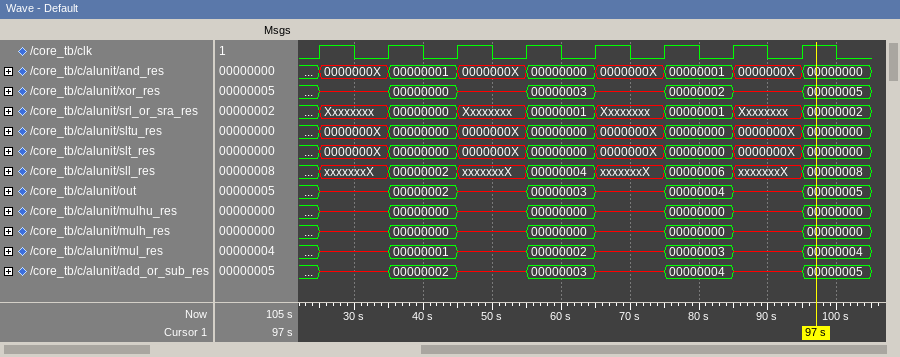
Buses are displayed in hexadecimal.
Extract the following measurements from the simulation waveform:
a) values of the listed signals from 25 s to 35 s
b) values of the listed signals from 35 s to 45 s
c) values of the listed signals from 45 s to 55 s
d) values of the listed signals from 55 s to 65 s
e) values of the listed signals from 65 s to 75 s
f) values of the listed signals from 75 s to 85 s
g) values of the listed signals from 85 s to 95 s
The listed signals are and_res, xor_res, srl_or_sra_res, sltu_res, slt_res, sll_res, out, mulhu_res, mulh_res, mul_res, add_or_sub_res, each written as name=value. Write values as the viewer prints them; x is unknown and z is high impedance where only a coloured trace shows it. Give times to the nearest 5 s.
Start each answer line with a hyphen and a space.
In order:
- and_res=0000000X, xor_res=x, srl_or_sra_res=Xxxxxxxx, sltu_res=0000000X, slt_res=0000000X, sll_res=xxxxxxxX, out=x, mulhu_res=x, mulh_res=x, mul_res=x, add_or_sub_res=x
- and_res=00000001, xor_res=00000000, srl_or_sra_res=00000000, sltu_res=00000000, slt_res=00000000, sll_res=00000002, out=00000002, mulhu_res=00000000, mulh_res=00000000, mul_res=00000001, add_or_sub_res=00000002
- and_res=0000000X, xor_res=x, srl_or_sra_res=Xxxxxxxx, sltu_res=0000000X, slt_res=0000000X, sll_res=xxxxxxxX, out=x, mulhu_res=x, mulh_res=x, mul_res=x, add_or_sub_res=x
- and_res=00000000, xor_res=00000003, srl_or_sra_res=00000001, sltu_res=00000000, slt_res=00000000, sll_res=00000004, out=00000003, mulhu_res=00000000, mulh_res=00000000, mul_res=00000002, add_or_sub_res=00000003
- and_res=0000000X, xor_res=x, srl_or_sra_res=Xxxxxxxx, sltu_res=0000000X, slt_res=0000000X, sll_res=xxxxxxxX, out=x, mulhu_res=x, mulh_res=x, mul_res=x, add_or_sub_res=x
- and_res=00000001, xor_res=00000002, srl_or_sra_res=00000001, sltu_res=00000000, slt_res=00000000, sll_res=00000006, out=00000004, mulhu_res=00000000, mulh_res=00000000, mul_res=00000003, add_or_sub_res=00000004
- and_res=0000000X, xor_res=x, srl_or_sra_res=Xxxxxxxx, sltu_res=0000000X, slt_res=0000000X, sll_res=xxxxxxxX, out=x, mulhu_res=x, mulh_res=x, mul_res=x, add_or_sub_res=x
